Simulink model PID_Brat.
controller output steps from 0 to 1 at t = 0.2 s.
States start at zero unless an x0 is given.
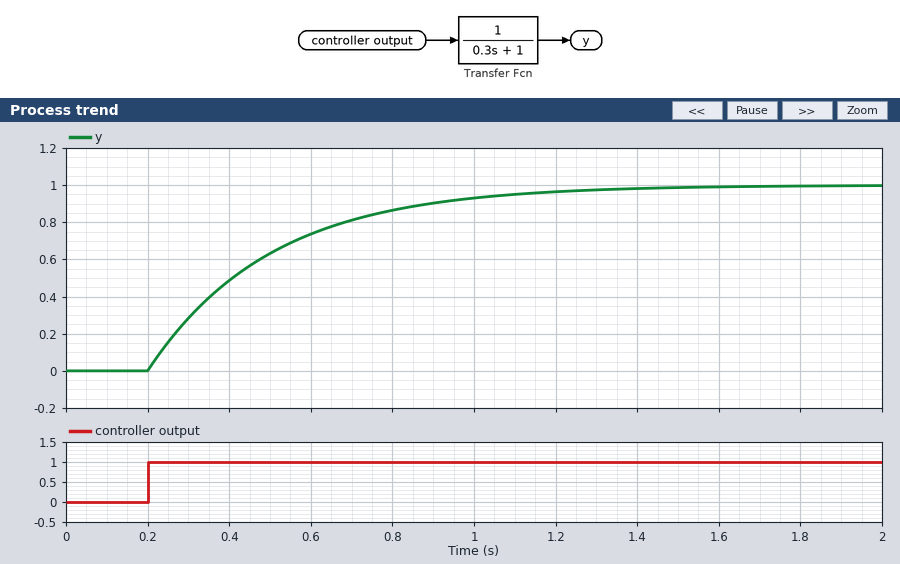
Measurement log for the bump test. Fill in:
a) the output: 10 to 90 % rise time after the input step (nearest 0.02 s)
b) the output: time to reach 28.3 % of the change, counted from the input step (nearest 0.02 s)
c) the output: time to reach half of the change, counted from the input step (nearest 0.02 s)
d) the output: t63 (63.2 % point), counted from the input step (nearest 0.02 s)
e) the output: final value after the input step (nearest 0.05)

0.66 s
0.10 s
0.20 s
0.30 s
1.00
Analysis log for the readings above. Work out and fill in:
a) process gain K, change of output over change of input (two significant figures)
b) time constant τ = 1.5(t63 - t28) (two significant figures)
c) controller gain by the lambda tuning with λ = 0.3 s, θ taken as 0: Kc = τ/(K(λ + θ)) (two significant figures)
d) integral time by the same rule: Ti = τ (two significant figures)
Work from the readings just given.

1.0
0.30 s
1.0
0.30 s
